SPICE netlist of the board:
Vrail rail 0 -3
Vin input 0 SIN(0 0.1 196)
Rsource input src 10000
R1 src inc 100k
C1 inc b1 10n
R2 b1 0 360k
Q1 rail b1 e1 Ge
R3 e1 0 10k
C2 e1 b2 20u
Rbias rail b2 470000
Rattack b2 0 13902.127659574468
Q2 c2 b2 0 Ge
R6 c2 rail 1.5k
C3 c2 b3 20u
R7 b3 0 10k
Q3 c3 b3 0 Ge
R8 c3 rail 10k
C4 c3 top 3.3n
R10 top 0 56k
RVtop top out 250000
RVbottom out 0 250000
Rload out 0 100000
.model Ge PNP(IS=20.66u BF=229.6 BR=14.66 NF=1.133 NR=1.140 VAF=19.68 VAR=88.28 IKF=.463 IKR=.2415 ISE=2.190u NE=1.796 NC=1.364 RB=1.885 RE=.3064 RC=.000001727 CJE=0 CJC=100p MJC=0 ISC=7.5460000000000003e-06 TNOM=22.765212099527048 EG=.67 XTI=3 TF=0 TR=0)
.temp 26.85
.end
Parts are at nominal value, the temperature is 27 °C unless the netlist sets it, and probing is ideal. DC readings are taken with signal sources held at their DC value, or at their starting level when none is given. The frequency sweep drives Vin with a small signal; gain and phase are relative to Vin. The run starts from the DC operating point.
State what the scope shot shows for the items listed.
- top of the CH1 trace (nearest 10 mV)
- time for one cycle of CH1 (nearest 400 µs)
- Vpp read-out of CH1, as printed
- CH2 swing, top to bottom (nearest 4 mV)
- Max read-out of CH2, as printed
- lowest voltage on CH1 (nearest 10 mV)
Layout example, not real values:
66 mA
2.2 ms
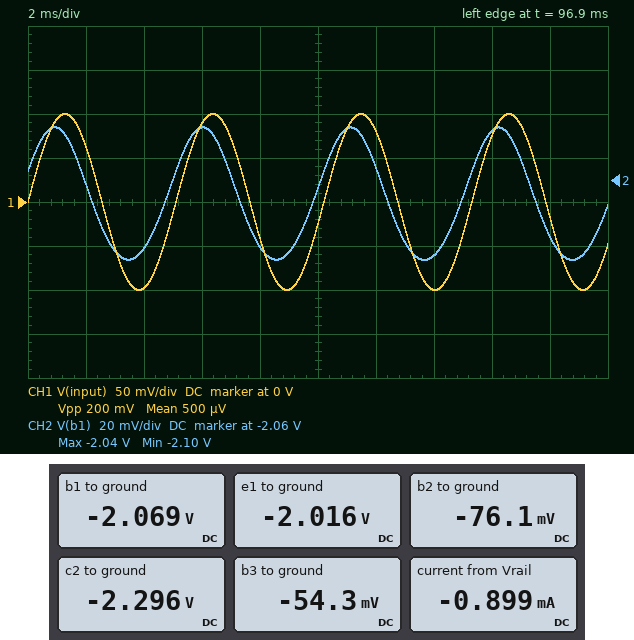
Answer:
100 mV
5.2 ms
200 mV
60 mV
-2.04 V
-100 mV
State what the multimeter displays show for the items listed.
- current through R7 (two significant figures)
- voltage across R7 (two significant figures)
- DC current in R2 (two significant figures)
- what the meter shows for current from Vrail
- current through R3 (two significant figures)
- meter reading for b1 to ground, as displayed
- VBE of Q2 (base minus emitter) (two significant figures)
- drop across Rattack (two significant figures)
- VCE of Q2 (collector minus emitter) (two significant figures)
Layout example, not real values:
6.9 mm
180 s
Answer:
5.4 µA
54 mV
5.7 µA
-0.899 mA
200 µA
-2.069 V
-76 mV
76 mV
-2.3 V
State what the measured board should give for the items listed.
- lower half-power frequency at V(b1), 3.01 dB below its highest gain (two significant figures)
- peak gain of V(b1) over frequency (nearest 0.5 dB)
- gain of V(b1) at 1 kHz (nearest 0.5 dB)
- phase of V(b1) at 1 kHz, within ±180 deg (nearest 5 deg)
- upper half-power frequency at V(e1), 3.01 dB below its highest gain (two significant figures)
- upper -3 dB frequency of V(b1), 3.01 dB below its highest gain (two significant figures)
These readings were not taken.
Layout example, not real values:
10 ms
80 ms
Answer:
96 Hz
-9.5 dB
-9.5 dB
5 deg
30 kHz
31 kHz
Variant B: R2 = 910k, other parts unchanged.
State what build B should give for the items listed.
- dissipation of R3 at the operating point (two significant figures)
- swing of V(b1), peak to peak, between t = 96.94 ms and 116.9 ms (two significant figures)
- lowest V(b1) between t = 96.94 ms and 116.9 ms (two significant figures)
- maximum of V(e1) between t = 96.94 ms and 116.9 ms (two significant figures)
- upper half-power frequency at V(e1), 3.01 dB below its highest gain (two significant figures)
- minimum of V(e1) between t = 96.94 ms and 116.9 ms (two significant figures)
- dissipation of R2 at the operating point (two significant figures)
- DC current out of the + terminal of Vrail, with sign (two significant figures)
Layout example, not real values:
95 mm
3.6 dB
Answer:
770 µW
60 mV
-2.9 V
-2.7 V
31 kHz
-2.8 V
8.8 µW
-970 µA
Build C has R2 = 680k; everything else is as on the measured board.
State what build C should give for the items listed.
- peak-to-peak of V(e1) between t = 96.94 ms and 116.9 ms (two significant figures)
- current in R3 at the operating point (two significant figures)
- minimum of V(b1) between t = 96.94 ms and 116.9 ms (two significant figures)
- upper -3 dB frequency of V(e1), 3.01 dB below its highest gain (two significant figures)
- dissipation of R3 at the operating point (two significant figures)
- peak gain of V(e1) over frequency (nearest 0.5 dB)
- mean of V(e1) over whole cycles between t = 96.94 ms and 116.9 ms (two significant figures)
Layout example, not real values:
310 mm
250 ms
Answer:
61 mV
260 µA
-2.7 V
28 kHz
660 µW
-9.5 dB
-2.6 V
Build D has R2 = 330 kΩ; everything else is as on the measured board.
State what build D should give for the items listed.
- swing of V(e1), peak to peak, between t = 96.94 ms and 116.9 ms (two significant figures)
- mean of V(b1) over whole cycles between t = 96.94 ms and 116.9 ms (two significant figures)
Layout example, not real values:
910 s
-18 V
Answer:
55 mV
-2.0 V
